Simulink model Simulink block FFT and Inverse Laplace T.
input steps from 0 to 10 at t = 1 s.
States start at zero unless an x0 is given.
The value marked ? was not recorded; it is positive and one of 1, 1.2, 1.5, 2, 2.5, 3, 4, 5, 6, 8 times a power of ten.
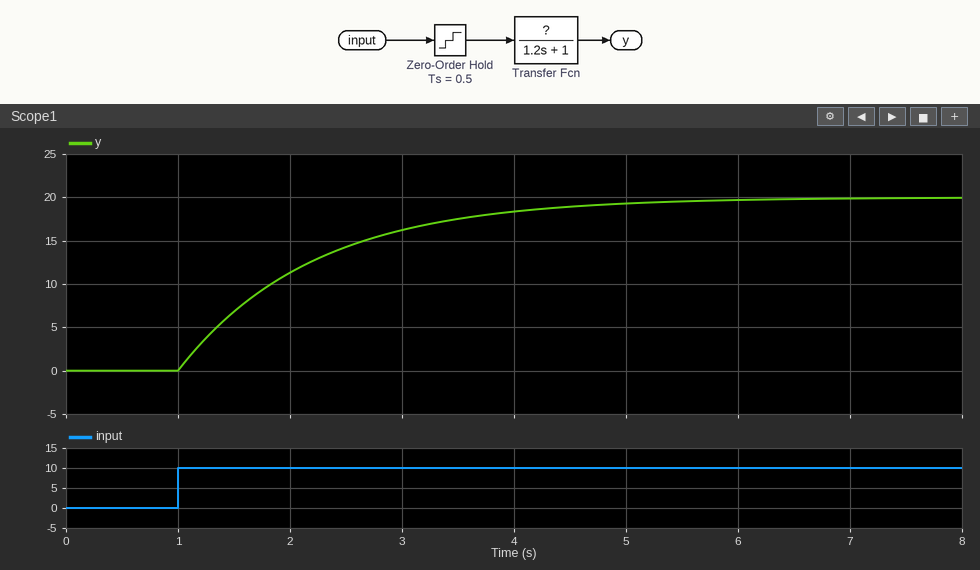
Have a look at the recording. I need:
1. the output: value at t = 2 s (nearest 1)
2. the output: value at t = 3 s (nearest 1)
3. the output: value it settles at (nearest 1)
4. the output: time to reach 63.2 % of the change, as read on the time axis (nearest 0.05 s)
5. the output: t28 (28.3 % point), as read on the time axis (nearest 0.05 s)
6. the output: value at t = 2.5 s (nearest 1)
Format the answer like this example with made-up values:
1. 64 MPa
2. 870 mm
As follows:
1. 11
2. 16
3. 20
4. 2.20 s
5. 1.40 s
6. 14
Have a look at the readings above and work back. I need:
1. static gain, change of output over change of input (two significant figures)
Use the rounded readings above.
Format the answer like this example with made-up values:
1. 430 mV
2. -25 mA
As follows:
1. 2.0
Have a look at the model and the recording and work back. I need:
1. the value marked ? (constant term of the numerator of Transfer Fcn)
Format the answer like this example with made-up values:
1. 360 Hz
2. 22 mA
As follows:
1. 2
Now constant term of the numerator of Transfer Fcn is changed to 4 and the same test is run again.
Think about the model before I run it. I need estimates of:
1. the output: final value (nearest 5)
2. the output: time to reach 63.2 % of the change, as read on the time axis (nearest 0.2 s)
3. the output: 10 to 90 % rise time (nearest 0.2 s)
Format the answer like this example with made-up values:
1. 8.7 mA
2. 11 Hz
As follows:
1. 40
2. 2.2 s
3. 2.6 s
